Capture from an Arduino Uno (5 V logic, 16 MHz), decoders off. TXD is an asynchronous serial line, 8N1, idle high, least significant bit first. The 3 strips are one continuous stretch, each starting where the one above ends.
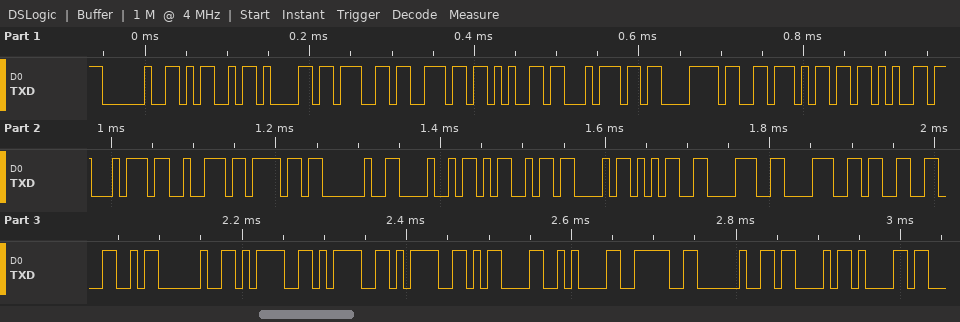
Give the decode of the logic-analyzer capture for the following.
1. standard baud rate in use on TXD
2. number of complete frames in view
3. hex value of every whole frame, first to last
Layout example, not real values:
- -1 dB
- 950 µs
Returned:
- 115200 baud
- 33
- 0x20 0x4D 0x61 0x67 0x6E 0x65 0x74 0xC3 0xB3 0x6D 0x65 0x74 0x72 0x6F 0x20 0x48 0x4D 0x43 0x35 0x38 0x38 0x33 0x4C 0x20 0x3D 0x3D 0x3D 0x0D 0x0A 0x3E 0x20 0x43 0x61
